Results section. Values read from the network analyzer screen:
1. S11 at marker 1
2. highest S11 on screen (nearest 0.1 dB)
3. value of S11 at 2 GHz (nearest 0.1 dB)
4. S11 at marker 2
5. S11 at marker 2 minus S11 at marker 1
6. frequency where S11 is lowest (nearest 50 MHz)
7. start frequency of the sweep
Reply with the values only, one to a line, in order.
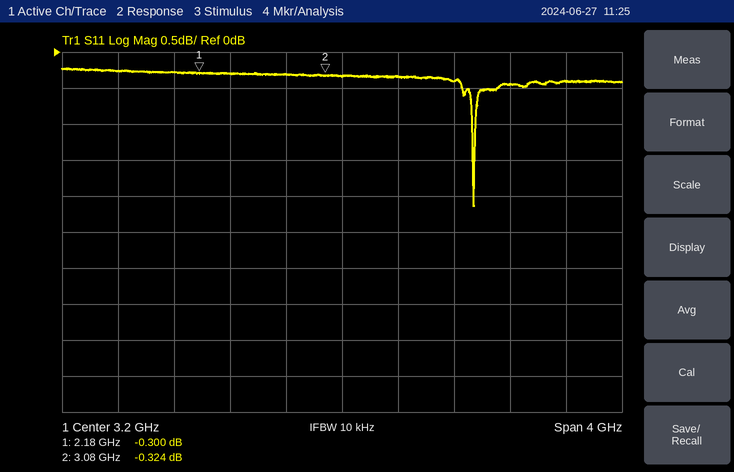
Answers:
-0.300 dB
-0.2 dB
-0.3 dB
-0.324 dB
-0.024 dB
4.15 GHz
1.2 GHz
